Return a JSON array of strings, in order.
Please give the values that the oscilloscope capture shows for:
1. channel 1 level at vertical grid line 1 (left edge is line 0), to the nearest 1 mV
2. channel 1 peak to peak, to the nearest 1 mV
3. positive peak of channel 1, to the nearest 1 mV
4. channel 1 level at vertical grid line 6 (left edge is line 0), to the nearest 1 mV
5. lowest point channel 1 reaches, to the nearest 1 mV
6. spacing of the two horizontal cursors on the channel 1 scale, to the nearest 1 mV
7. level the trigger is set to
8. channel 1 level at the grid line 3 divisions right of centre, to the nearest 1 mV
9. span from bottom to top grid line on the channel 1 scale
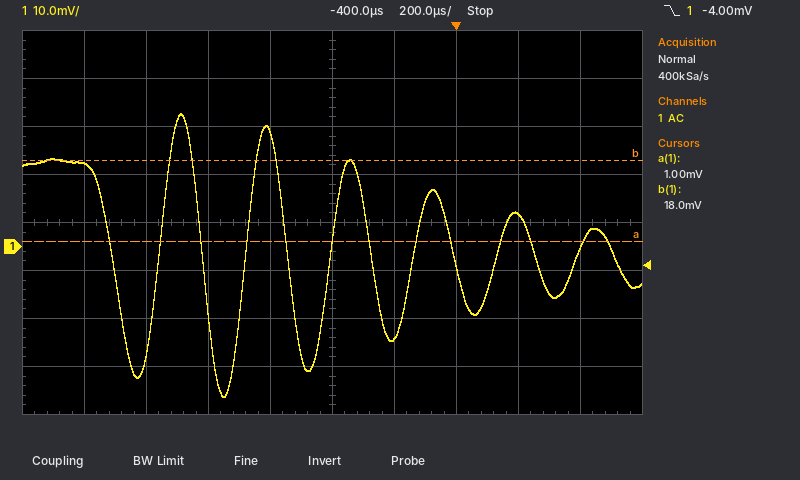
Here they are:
["17 mV", "59 mV", "28 mV", "-19 mV", "-31 mV", "17 mV", "-4.00 mV", "7 mV", "80 mV"]
